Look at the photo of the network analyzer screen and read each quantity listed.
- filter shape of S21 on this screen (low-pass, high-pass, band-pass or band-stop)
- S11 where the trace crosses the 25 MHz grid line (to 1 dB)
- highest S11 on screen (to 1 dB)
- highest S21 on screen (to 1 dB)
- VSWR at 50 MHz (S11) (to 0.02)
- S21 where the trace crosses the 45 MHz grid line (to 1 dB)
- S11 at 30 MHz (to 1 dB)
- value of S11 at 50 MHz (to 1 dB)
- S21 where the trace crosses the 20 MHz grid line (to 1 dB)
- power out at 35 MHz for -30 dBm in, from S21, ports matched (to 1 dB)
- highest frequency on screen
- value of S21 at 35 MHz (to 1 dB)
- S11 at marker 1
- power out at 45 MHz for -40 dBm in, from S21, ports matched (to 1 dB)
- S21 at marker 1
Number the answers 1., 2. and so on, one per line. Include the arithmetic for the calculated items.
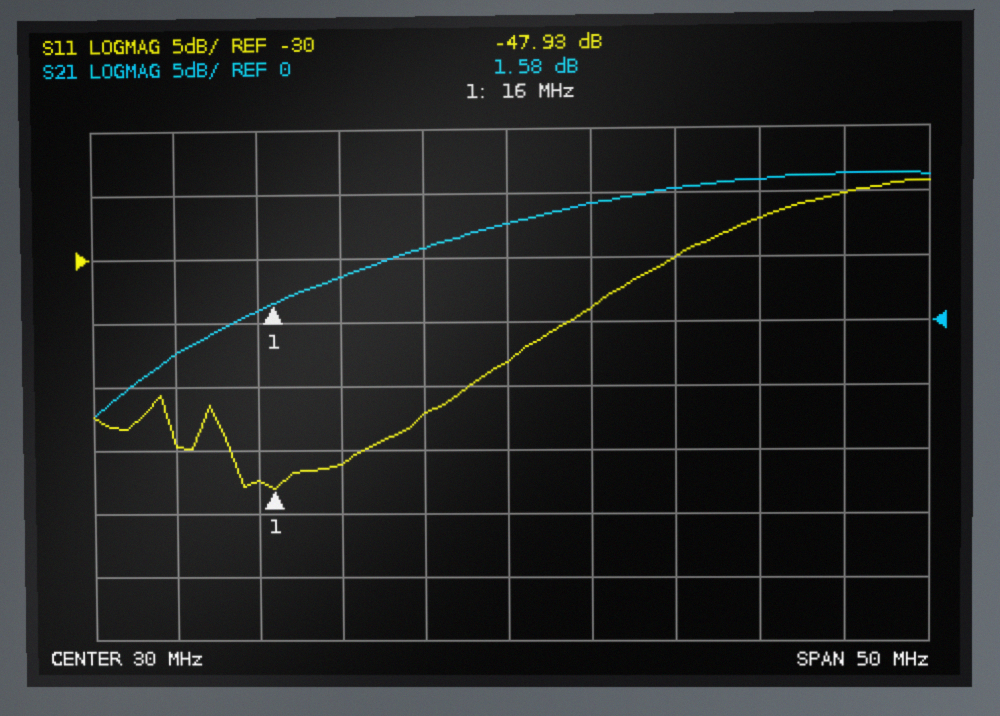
1. high-pass
2. -42 dB
3. -24 dB
4. 11 dB
5. |Γ| = 10^(-25/20) = 0.0562; VSWR = (1 + 0.0562)/(1 − 0.0562) ≈ 1.12
6. 11 dB
7. -38 dB
8. -25 dB
9. 4 dB
10. -30 dBm + (9 dB) = -21 dBm
11. 55 MHz
12. 9 dB
13. -47.93 dB
14. -40 dBm + (11 dB) = -29 dBm
15. 1.58 dB
